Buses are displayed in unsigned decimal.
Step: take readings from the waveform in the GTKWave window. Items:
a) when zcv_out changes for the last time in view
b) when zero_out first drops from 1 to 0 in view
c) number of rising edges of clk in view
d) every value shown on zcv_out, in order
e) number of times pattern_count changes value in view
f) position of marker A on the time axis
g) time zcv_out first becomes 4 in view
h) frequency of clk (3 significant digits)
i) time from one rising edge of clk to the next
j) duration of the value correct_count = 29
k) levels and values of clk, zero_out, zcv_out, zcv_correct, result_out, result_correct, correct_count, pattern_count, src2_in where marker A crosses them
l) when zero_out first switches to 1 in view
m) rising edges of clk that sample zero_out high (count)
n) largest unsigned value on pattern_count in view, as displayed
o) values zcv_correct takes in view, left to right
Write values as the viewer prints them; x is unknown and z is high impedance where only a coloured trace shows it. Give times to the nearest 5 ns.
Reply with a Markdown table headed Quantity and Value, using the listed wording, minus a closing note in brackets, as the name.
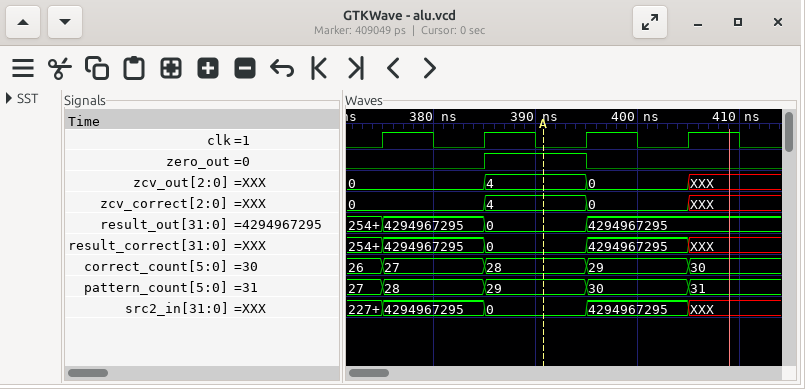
| Quantity | Value |
|---|---|
| when zcv_out changes for the last time in view | 405 ns |
| when zero_out first drops from 1 to 0 in view | 395 ns |
| number of rising edges of clk in view | 4 |
| every value shown on zcv_out, in order | 0, 4, 0, XXX |
| number of times pattern_count changes value in view | 4 |
| position of marker A on the time axis | 390 ns |
| time zcv_out first becomes 4 in view | 385 ns |
| frequency of clk | 100 MHz |
| time from one rising edge of clk to the next | 10 ns |
| duration of the value correct_count = 29 | 10 ns |
| levels and values of clk, zero_out, zcv_out, zcv_correct, result_out, result_correct, correct_count, pattern_count, src2_in where marker A crosses them | clk=0, zero_out=1, zcv_out=4, zcv_correct=4, result_out=0, result_correct=0, correct_count=28, pattern_count=29, src2_in=0 |
| when zero_out first switches to 1 in view | 385 ns |
| rising edges of clk that sample zero_out high | 1 |
| largest unsigned value on pattern_count in view, as displayed | 31 |
| values zcv_correct takes in view, left to right | 0, 4, 0, XXX |
